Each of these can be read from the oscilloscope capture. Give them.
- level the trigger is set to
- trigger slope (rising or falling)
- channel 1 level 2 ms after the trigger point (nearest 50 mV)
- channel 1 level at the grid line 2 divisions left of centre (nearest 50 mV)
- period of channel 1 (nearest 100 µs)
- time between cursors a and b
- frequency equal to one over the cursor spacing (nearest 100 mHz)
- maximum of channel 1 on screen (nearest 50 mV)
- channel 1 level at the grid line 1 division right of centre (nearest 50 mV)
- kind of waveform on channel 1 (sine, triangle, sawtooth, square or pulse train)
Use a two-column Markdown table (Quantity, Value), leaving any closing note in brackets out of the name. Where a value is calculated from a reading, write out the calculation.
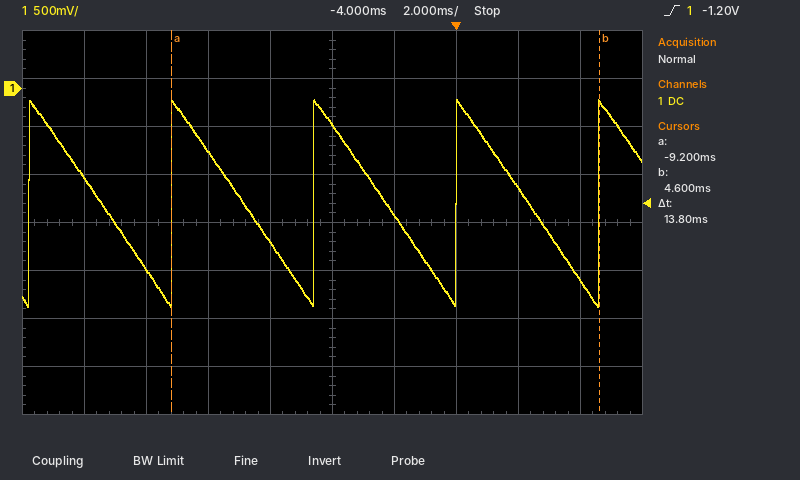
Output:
| Quantity | Value |
|---|---|
| level the trigger is set to | -1.20 V |
| trigger slope | rising |
| channel 1 level 2 ms after the trigger point | -1.05 V |
| channel 1 level at the grid line 2 divisions left of centre | -650 mV |
| period of channel 1 | 4.6 ms |
| time between cursors a and b | 13.8 ms |
| frequency equal to one over the cursor spacing | 1 / 13.8 ms ≈ 72.5 Hz |
| maximum of channel 1 on screen | -100 mV |
| channel 1 level at the grid line 1 division right of centre | -1.30 V |
| kind of waveform on channel 1 | sawtooth |
